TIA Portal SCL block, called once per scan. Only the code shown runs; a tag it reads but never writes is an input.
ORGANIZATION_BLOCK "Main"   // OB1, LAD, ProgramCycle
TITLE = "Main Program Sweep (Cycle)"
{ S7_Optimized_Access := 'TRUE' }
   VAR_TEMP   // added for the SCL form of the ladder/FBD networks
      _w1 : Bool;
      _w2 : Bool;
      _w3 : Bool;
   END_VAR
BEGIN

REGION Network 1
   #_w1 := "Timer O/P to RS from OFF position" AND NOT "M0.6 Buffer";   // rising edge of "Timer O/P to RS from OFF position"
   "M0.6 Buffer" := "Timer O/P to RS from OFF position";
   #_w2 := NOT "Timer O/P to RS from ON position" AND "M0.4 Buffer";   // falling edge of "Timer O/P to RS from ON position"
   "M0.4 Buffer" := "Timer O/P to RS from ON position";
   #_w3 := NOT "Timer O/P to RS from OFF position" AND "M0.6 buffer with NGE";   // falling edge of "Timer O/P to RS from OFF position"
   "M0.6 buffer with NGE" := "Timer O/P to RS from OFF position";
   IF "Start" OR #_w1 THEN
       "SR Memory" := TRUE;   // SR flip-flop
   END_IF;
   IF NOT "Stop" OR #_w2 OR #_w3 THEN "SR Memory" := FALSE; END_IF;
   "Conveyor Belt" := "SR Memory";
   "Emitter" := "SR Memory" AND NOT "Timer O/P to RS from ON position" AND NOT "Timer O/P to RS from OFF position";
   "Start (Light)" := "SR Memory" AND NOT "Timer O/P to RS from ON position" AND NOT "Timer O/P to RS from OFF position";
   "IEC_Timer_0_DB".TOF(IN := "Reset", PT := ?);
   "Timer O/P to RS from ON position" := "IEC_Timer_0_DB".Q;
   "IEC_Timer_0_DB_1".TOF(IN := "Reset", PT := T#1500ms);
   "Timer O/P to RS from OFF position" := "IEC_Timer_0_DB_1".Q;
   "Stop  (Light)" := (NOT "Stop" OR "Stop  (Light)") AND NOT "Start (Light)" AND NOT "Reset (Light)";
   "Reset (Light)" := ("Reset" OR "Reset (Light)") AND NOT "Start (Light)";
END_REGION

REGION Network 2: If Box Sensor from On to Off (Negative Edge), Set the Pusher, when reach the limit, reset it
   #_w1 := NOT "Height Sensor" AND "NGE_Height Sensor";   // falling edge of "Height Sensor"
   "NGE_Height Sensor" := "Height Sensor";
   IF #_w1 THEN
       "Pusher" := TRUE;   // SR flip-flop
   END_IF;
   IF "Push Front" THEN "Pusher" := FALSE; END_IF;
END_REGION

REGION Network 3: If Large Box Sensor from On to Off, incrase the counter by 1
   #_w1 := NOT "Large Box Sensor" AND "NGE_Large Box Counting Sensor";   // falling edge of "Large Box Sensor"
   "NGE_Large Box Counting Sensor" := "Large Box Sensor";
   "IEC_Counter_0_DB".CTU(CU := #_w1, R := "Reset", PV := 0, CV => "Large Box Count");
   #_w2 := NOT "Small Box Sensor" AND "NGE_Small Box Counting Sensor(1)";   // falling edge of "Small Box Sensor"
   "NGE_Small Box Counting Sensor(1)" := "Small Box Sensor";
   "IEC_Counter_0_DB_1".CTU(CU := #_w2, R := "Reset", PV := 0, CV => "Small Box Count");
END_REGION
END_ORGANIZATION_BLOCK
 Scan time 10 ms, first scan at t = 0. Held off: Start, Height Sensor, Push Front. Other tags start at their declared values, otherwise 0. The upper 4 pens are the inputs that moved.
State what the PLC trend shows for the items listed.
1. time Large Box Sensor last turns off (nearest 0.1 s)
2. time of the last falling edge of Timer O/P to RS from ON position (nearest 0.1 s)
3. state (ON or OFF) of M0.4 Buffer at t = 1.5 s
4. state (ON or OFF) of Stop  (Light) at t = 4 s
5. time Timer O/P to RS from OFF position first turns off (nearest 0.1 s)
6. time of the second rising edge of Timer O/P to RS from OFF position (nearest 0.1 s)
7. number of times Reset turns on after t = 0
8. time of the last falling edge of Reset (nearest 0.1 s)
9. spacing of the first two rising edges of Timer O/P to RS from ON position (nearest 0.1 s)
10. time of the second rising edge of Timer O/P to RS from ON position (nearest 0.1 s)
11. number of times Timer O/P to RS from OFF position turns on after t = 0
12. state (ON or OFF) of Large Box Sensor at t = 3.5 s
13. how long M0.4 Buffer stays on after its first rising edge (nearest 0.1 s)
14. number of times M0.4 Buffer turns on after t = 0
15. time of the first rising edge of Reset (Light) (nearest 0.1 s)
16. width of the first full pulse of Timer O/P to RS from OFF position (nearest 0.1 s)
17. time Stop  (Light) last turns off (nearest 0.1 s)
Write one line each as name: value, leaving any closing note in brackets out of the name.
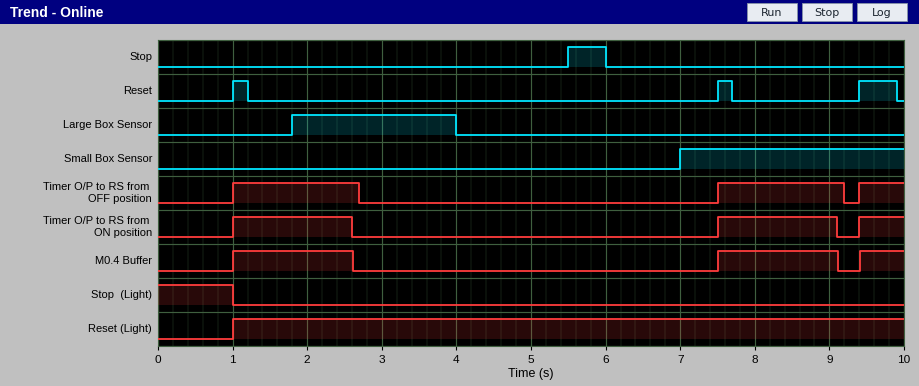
time Large Box Sensor last turns off: 4.0 s
time of the last falling edge of Timer O/P to RS from ON position: 9.1 s
state (ON or OFF) of M0.4 Buffer at t = 1.5 s: ON
state (ON or OFF) of Stop  (Light) at t = 4 s: OFF
time Timer O/P to RS from OFF position first turns off: 2.7 s
time of the second rising edge of Timer O/P to RS from OFF position: 7.5 s
number of times Reset turns on after t = 0: 3
time of the last falling edge of Reset: 9.9 s
spacing of the first two rising edges of Timer O/P to RS from ON position: 6.5 s
time of the second rising edge of Timer O/P to RS from ON position: 7.5 s
number of times Timer O/P to RS from OFF position turns on after t = 0: 3
state (ON or OFF) of Large Box Sensor at t = 3.5 s: ON
how long M0.4 Buffer stays on after its first rising edge: 1.6 s
number of times M0.4 Buffer turns on after t = 0: 3
time of the first rising edge of Reset (Light): 1.0 s
width of the first full pulse of Timer O/P to RS from OFF position: 1.7 s
time Stop  (Light) last turns off: 1.0 s
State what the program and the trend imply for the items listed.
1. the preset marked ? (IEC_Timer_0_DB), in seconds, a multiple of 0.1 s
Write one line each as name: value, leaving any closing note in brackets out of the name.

the preset marked ? (IEC_Timer_0_DB), in seconds, a multiple of 0.1 s: 1.4 s
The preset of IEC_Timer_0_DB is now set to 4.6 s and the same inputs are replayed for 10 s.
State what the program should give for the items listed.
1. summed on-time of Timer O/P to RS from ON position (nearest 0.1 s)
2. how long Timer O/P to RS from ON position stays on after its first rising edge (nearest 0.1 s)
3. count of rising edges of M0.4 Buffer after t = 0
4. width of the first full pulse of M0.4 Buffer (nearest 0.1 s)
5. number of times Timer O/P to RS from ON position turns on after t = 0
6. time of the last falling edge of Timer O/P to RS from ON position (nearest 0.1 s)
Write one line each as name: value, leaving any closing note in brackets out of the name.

summed on-time of Timer O/P to RS from ON position: 7.3 s
how long Timer O/P to RS from ON position stays on after its first rising edge: 4.8 s
count of rising edges of M0.4 Buffer after t = 0: 2
width of the first full pulse of M0.4 Buffer: 4.8 s
number of times Timer O/P to RS from ON position turns on after t = 0: 2
time of the last falling edge of Timer O/P to RS from ON position: 5.8 s
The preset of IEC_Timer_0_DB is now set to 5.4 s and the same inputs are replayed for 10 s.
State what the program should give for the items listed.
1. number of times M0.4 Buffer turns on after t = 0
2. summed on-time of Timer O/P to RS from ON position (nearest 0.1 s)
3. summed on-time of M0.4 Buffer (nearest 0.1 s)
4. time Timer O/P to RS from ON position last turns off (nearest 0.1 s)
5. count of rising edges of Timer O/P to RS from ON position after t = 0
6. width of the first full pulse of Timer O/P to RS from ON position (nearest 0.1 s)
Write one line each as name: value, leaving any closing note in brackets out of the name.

number of times M0.4 Buffer turns on after t = 0: 2
summed on-time of Timer O/P to RS from ON position: 8.1 s
summed on-time of M0.4 Buffer: 8.1 s
time Timer O/P to RS from ON position last turns off: 6.6 s
count of rising edges of Timer O/P to RS from ON position after t = 0: 2
width of the first full pulse of Timer O/P to RS from ON position: 5.6 s
